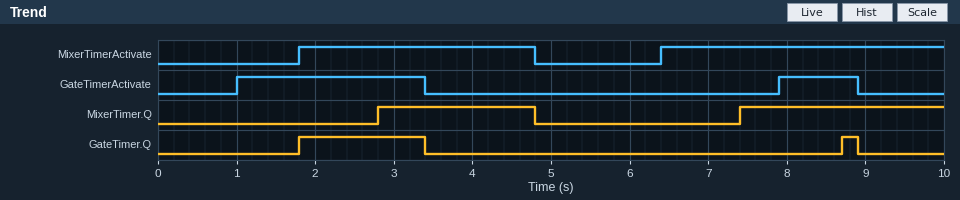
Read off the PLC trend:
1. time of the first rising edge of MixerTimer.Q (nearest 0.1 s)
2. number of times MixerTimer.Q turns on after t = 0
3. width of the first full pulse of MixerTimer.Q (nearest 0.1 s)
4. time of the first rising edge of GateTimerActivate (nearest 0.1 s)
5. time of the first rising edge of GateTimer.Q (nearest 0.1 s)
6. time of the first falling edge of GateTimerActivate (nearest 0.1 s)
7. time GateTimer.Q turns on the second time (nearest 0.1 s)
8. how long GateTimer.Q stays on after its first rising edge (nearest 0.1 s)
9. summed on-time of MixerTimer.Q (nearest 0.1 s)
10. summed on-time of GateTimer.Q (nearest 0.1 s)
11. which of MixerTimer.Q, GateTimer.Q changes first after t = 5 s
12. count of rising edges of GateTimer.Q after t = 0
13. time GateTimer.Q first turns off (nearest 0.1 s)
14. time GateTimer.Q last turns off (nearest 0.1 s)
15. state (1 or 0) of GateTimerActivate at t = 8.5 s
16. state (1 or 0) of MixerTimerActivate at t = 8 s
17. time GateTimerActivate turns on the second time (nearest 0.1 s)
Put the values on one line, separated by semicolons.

2.8 s; 2; 2.0 s; 1.0 s; 1.8 s; 3.4 s; 8.7 s; 1.6 s; 4.6 s; 1.8 s; MixerTimer.Q; 2; 3.4 s; 8.9 s; 1; 1; 7.9 s
